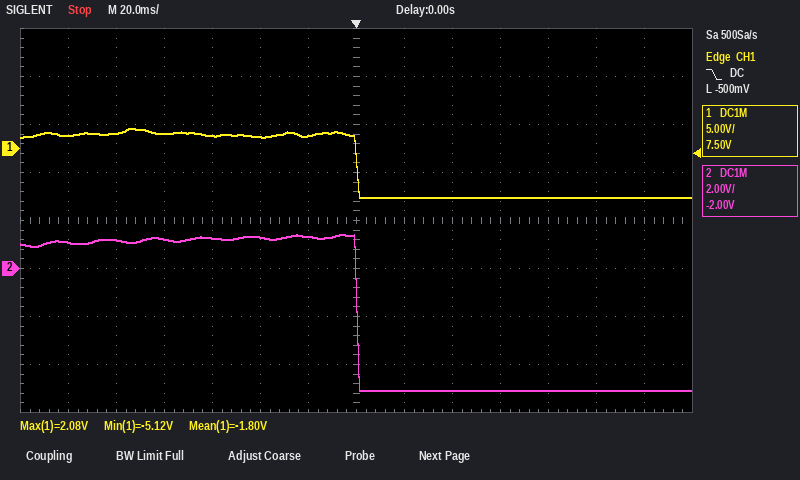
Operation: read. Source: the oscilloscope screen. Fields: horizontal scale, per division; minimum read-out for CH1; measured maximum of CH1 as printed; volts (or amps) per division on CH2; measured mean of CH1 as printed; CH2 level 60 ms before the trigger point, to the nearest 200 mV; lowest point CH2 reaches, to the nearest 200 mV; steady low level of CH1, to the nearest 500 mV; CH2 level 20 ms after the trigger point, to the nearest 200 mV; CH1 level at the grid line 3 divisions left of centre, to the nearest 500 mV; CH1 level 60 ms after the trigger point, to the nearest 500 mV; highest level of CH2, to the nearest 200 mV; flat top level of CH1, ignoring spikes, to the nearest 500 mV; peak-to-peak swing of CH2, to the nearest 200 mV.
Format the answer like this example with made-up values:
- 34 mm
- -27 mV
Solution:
- 20 ms
- -5.12 V
- 2.08 V
- 2 V
- -1.80 V
- 1.2 V
- -5.0 V
- -5.0 V
- -5.0 V
- 1.5 V
- -5.0 V
- 1.4 V
- 1.5 V
- 6.4 V
